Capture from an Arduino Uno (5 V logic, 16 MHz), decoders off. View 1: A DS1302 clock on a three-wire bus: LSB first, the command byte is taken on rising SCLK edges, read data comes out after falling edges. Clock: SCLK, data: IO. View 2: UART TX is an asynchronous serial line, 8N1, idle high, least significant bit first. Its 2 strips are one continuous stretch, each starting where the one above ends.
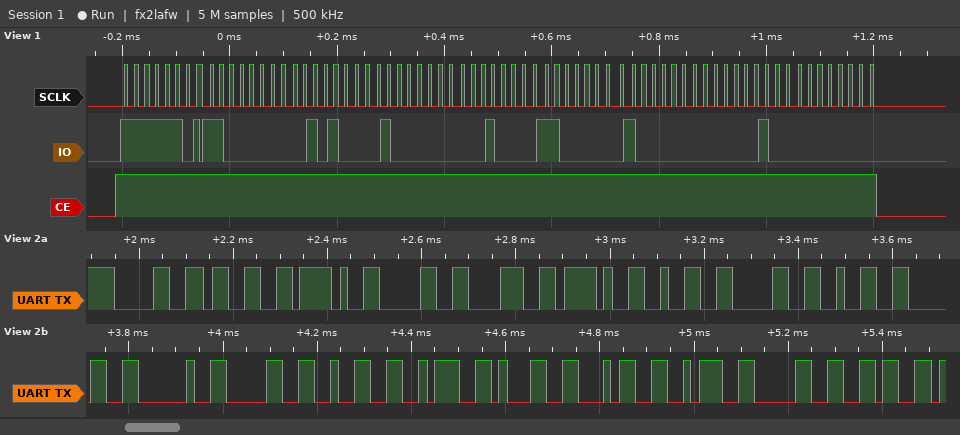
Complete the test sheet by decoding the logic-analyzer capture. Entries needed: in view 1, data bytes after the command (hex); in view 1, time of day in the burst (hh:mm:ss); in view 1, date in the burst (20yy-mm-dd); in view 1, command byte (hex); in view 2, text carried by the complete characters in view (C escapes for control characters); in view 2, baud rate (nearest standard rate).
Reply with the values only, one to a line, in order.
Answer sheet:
03 14 02 08 03 01 20 00
02:14:03
2020-03-08
0xBF
"03/08/2020 02:14:06"
57600 baud
